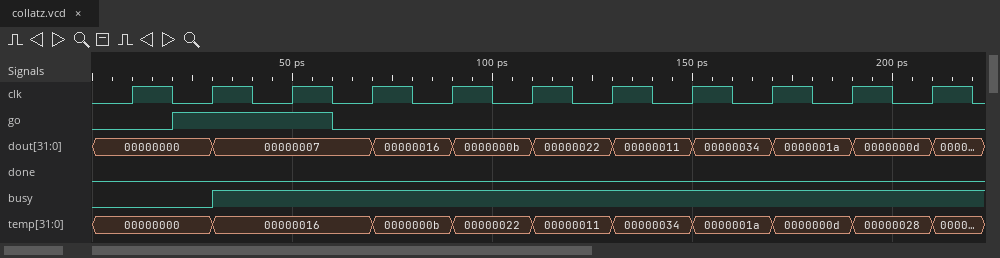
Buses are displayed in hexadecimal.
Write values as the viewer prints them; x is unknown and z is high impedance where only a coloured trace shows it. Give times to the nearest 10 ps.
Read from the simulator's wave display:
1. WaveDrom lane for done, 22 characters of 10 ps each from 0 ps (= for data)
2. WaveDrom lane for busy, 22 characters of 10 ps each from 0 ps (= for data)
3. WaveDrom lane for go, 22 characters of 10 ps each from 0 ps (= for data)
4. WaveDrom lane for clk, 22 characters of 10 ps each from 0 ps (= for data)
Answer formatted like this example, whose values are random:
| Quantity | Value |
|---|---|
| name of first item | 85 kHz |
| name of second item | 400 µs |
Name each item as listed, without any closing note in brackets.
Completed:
| Quantity | Value |
|---|---|
| WaveDrom lane for done, 22 characters of 10 ps each from 0 ps | {name: 'done', wave: '0.....................'} |
| WaveDrom lane for busy, 22 characters of 10 ps each from 0 ps | {name: 'busy', wave: '0..1..................'} |
| WaveDrom lane for go, 22 characters of 10 ps each from 0 ps | {name: 'go', wave: '0.1...0...............'} |
| WaveDrom lane for clk, 22 characters of 10 ps each from 0 ps | {name: 'clk', wave: '0101010101010101010101'} |
